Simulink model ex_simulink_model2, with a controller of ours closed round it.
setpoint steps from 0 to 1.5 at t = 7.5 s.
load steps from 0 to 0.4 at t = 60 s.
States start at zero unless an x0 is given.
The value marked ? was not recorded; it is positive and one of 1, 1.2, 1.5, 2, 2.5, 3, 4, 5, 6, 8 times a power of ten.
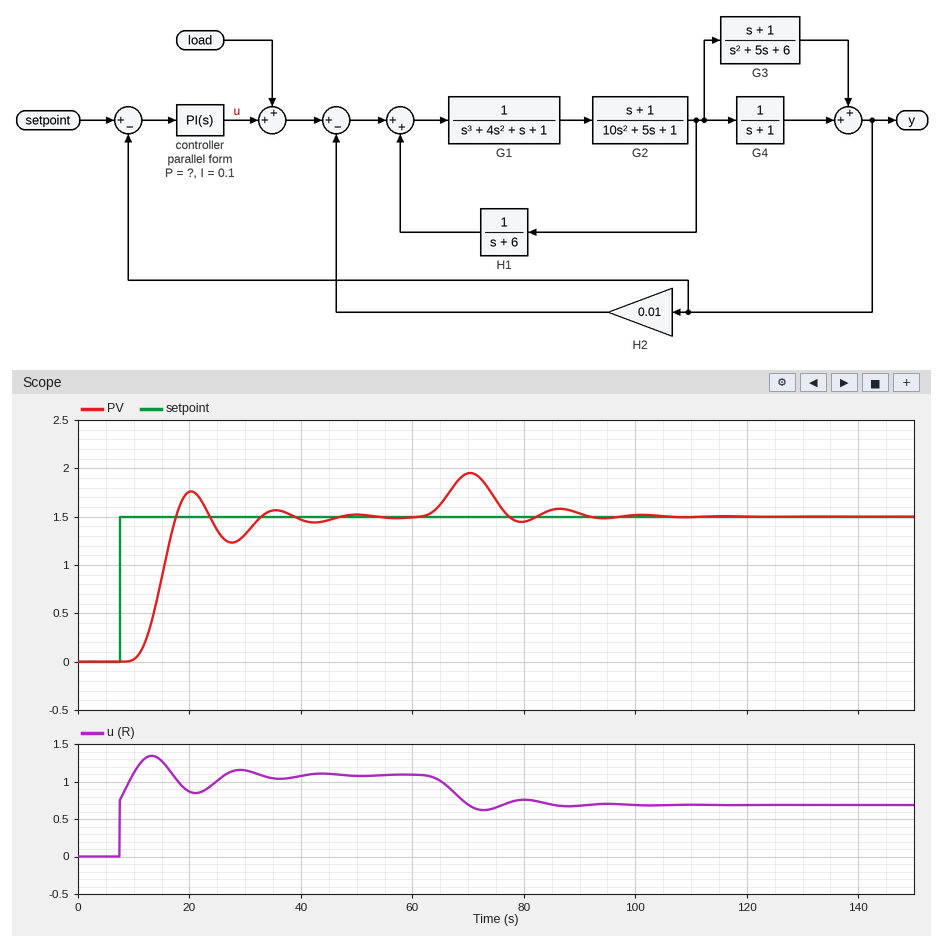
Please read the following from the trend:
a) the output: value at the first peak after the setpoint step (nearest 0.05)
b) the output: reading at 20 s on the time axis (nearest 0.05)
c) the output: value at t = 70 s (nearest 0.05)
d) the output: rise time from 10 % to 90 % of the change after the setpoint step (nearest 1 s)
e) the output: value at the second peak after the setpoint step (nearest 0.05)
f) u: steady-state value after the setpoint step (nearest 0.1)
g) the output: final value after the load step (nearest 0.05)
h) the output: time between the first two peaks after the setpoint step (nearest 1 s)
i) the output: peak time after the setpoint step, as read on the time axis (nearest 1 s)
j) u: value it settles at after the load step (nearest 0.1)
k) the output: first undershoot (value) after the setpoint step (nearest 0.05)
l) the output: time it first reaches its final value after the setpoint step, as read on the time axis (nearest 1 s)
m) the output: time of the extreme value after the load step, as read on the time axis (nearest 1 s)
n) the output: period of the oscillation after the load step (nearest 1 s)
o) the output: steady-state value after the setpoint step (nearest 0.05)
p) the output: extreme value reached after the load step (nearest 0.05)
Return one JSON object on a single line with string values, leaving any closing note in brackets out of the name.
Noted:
{"the output: value at the first peak after the setpoint step": "1.75", "the output: reading at 20 s on the time axis": "1.75", "the output: value at t = 70 s": "1.95", "the output: rise time from 10 % to 90 % of the change after the setpoint step": "5 s", "the output: value at the second peak after the setpoint step": "1.55", "u: steady-state value after the setpoint step": "1.1", "the output: final value after the load step": "1.50", "the output: time between the first two peaks after the setpoint step": "15 s", "the output: peak time after the setpoint step, as read on the time axis": "20 s", "u: value it settles at after the load step": "0.7", "the output: first undershoot (value) after the setpoint step": "1.25", "the output: time it first reaches its final value after the setpoint step, as read on the time axis": "18 s", "the output: time of the extreme value after the load step, as read on the time axis": "70 s", "the output: period of the oscillation after the load step": "16 s", "the output: steady-state value after the setpoint step": "1.50", "the output: extreme value reached after the load step": "1.95"}
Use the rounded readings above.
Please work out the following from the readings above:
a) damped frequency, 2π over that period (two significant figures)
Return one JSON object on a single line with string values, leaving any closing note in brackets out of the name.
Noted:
{"damped frequency, 2π over that period": "0.42 rad/s"}
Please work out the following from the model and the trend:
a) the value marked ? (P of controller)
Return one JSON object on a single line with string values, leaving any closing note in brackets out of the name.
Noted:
{"the value marked ?": "0.5"}
